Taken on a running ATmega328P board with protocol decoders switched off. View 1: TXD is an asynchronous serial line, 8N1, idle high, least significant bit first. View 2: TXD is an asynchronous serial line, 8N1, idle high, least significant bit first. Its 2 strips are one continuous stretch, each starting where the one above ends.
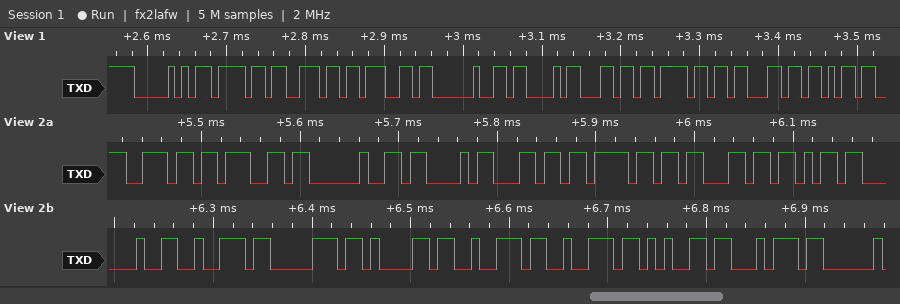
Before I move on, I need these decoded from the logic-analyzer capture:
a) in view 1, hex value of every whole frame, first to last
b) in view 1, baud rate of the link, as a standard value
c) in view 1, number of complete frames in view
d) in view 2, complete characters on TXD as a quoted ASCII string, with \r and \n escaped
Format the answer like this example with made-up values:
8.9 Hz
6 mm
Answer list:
50 6F 6E 67 20 43 6C 6F 63 6B
115200 baud
10
"ng Clock rparret"
